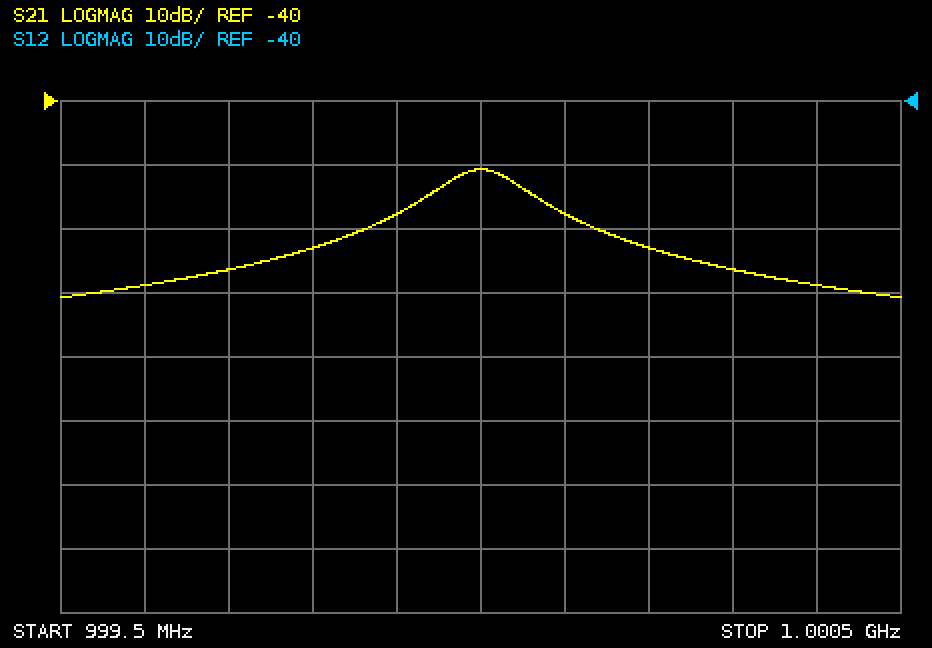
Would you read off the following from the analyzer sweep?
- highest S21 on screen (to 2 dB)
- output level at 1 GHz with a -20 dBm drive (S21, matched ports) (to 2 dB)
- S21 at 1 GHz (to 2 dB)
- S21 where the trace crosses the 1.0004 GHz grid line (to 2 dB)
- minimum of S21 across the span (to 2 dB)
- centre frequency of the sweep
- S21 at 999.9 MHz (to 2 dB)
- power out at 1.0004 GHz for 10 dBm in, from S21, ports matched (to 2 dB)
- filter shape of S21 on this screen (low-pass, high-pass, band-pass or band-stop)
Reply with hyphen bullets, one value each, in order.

- -50 dB
- -70 dBm
- -50 dB
- -68 dB
- -70 dB
- 1 GHz
- -58 dB
- -58 dBm
- band-pass
